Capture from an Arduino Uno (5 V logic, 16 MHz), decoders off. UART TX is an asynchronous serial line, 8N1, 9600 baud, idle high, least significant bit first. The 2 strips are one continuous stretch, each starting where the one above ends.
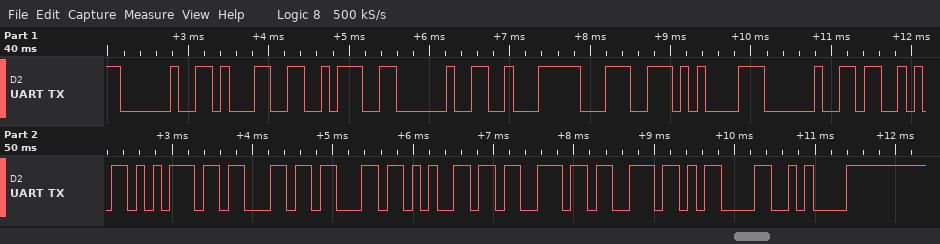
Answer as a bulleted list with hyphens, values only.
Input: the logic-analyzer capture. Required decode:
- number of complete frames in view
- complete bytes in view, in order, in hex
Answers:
- 17
- 20 31 3A 20 E2 9C 85 20 53 75 63 63 65 73 73 0D 0A
